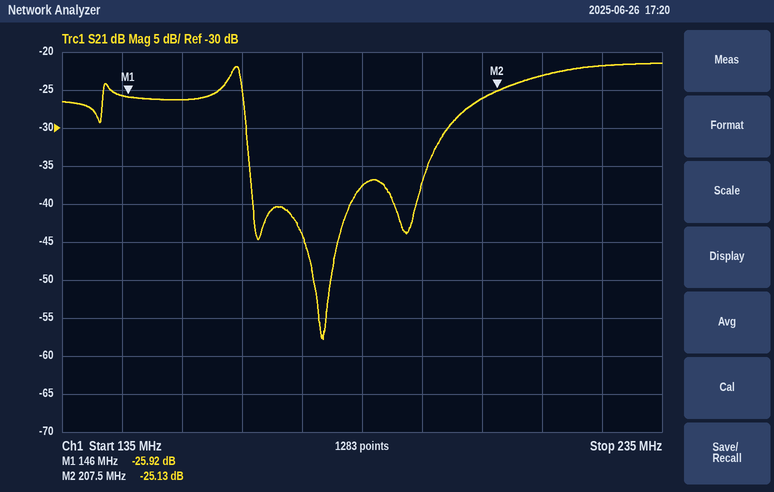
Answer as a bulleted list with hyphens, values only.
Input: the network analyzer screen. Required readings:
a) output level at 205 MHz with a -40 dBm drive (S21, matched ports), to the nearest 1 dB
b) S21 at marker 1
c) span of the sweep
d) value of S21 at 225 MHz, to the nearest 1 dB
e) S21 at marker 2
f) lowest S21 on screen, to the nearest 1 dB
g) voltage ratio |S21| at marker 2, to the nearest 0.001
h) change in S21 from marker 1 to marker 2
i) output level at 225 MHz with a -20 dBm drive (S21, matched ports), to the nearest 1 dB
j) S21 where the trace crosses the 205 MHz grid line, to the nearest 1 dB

- -66 dBm
- -25.92 dB
- 100 MHz
- -22 dB
- -25.13 dB
- -58 dB
- 0.055
- 0.79 dB
- -42 dBm
- -26 dB
